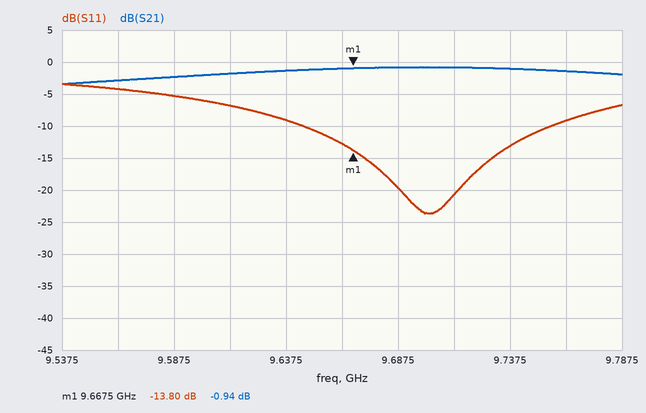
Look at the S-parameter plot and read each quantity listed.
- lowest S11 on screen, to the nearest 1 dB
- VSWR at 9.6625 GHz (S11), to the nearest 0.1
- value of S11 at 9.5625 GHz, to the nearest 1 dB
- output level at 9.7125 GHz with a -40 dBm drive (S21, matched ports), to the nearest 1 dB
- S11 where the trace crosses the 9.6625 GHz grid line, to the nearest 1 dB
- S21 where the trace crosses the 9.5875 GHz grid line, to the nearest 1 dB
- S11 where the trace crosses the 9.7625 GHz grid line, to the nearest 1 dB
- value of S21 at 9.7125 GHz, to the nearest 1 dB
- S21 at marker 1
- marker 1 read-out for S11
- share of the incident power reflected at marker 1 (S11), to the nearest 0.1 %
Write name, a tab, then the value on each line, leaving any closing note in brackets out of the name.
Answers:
lowest S11 on screen, to the nearest 1 dB	-24 dB
VSWR at 9.6625 GHz (S11), to the nearest 0.1	1.6
value of S11 at 9.5625 GHz, to the nearest 1 dB	-4 dB
output level at 9.7125 GHz with a -40 dBm drive (S21, matched ports), to the nearest 1 dB	-41 dBm
S11 where the trace crosses the 9.6625 GHz grid line, to the nearest 1 dB	-13 dB
S21 where the trace crosses the 9.5875 GHz grid line, to the nearest 1 dB	-2 dB
S11 where the trace crosses the 9.7625 GHz grid line, to the nearest 1 dB	-9 dB
value of S21 at 9.7125 GHz, to the nearest 1 dB	-1 dB
S21 at marker 1	-0.94 dB
marker 1 read-out for S11	-13.80 dB
share of the incident power reflected at marker 1 (S11), to the nearest 0.1 %	4.2 %
